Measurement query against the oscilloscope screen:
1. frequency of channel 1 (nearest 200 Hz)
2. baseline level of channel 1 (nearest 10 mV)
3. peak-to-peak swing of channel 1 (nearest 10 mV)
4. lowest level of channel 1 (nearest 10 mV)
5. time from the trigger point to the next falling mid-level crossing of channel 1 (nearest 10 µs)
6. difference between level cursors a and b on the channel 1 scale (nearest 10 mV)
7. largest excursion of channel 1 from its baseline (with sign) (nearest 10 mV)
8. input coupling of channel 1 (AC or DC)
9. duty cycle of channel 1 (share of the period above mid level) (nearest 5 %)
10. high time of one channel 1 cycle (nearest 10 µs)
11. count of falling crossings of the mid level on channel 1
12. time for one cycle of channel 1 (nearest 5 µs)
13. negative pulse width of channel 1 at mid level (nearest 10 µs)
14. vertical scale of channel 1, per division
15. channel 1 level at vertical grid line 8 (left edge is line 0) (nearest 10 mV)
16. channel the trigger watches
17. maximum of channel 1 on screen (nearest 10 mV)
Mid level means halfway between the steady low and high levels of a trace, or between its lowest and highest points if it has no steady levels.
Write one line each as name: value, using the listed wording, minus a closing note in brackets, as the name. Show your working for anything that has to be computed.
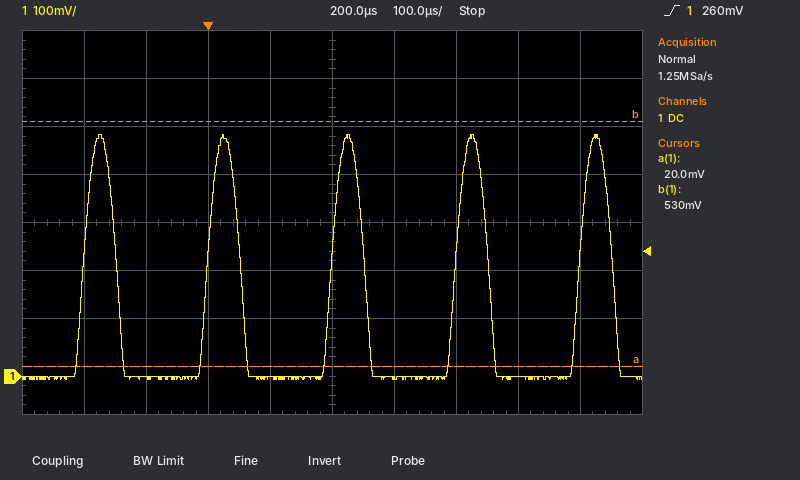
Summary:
frequency of channel 1: 1 / 200 µs ≈ 5.0 kHz
baseline level of channel 1: 0 mV
peak-to-peak swing of channel 1: 500 mV − (-10 mV) = 510 mV
lowest level of channel 1: -10 mV
time from the trigger point to the next falling mid-level crossing of channel 1: 50 µs
difference between level cursors a and b on the channel 1 scale: 510 mV
largest excursion of channel 1 from its baseline (with sign): 500 mV − (0 mV) = +500 mV
input coupling of channel 1: DC
duty cycle of channel 1 (share of the period above mid level): 50 µs / 200 µs ≈ 25 %
high time of one channel 1 cycle: 50 µs
count of falling crossings of the mid level on channel 1: 5
time for one cycle of channel 1: 200 µs
negative pulse width of channel 1 at mid level: 150 µs
vertical scale of channel 1, per division: 100 mV
channel 1 level at vertical grid line 8 (left edge is line 0): 0 mV
channel the trigger watches: channel 1
maximum of channel 1 on screen: 500 mV
